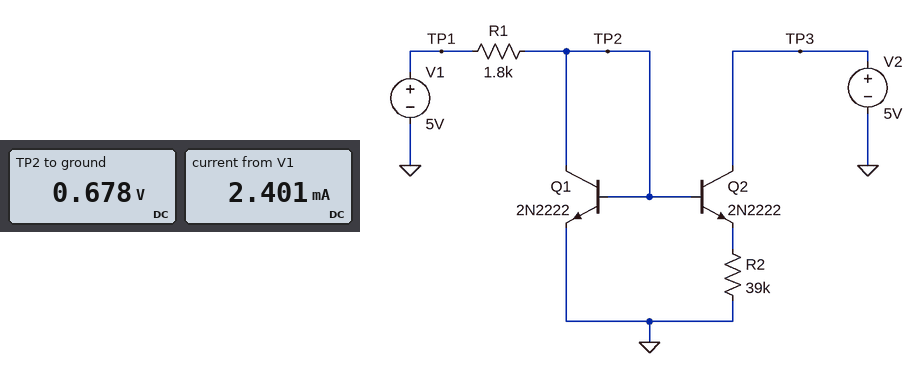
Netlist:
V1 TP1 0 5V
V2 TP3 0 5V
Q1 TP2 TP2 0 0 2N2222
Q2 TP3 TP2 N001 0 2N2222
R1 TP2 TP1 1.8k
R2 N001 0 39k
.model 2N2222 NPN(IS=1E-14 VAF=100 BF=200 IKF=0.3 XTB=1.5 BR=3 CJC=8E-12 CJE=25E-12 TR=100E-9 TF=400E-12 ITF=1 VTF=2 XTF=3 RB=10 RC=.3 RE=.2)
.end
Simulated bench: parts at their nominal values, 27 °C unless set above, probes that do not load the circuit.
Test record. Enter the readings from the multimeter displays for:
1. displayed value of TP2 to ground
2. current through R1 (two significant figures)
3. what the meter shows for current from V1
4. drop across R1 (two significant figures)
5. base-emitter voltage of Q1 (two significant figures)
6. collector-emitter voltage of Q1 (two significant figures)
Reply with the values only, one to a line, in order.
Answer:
0.678 V
2.4 mA
2.401 mA
4.3 V
680 mV
680 mV
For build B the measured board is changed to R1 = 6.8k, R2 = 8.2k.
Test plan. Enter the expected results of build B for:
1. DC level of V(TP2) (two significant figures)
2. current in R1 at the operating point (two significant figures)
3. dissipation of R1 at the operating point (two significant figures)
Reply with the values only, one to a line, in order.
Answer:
640 mV
640 µA
2.8 mW
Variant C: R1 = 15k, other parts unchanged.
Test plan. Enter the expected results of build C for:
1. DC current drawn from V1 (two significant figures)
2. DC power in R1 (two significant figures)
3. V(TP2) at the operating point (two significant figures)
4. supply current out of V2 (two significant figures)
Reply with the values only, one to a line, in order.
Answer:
290 µA
1.3 mW
620 mV
3.0 µA
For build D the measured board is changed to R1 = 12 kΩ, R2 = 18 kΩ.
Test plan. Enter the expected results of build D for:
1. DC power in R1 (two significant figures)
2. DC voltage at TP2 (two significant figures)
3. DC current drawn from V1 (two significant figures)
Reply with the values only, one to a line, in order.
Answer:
1.6 mW
630 mV
360 µA
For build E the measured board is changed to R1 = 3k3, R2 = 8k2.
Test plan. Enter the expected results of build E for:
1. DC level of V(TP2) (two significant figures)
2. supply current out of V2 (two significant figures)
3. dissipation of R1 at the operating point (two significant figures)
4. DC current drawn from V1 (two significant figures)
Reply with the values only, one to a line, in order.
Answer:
660 mV
14 µA
5.7 mW
1.3 mA
